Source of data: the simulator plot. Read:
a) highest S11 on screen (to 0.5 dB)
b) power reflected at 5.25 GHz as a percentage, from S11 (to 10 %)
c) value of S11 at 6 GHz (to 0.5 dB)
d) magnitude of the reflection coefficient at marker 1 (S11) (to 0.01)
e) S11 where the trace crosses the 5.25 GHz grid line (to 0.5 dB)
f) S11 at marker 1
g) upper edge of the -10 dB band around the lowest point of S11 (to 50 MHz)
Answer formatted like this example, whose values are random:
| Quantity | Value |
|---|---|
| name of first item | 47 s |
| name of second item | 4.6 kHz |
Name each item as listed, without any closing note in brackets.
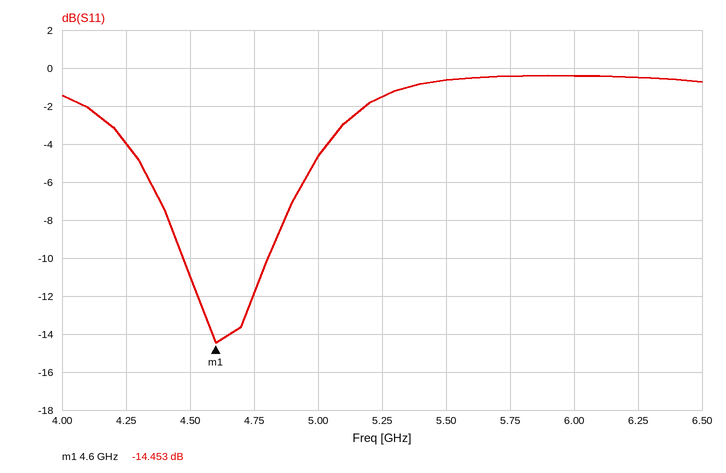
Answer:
| Quantity | Value |
|---|---|
| highest S11 on screen | -0.5 dB |
| power reflected at 5.25 GHz as a percentage, from S11 | 70 % |
| value of S11 at 6 GHz | -0.5 dB |
| magnitude of the reflection coefficient at marker 1 (S11) | 0.19 |
| S11 where the trace crosses the 5.25 GHz grid line | -1.5 dB |
| S11 at marker 1 | -14.453 dB |
| upper edge of the -10 dB band around the lowest point of S11 | 4.80 GHz |
